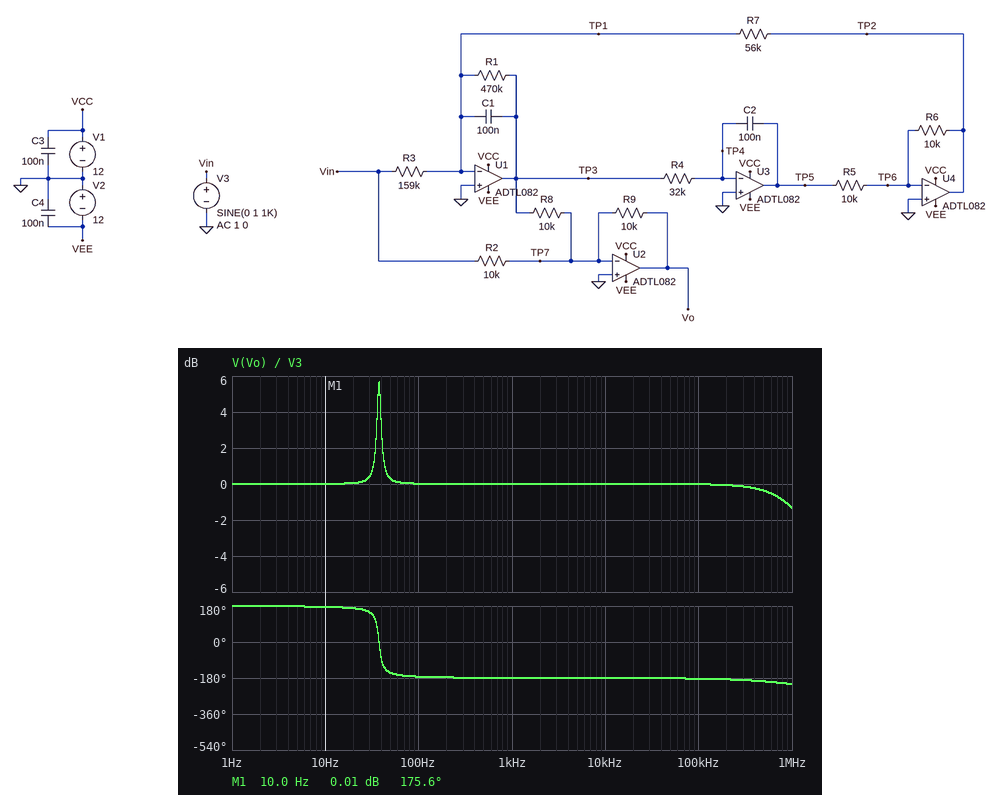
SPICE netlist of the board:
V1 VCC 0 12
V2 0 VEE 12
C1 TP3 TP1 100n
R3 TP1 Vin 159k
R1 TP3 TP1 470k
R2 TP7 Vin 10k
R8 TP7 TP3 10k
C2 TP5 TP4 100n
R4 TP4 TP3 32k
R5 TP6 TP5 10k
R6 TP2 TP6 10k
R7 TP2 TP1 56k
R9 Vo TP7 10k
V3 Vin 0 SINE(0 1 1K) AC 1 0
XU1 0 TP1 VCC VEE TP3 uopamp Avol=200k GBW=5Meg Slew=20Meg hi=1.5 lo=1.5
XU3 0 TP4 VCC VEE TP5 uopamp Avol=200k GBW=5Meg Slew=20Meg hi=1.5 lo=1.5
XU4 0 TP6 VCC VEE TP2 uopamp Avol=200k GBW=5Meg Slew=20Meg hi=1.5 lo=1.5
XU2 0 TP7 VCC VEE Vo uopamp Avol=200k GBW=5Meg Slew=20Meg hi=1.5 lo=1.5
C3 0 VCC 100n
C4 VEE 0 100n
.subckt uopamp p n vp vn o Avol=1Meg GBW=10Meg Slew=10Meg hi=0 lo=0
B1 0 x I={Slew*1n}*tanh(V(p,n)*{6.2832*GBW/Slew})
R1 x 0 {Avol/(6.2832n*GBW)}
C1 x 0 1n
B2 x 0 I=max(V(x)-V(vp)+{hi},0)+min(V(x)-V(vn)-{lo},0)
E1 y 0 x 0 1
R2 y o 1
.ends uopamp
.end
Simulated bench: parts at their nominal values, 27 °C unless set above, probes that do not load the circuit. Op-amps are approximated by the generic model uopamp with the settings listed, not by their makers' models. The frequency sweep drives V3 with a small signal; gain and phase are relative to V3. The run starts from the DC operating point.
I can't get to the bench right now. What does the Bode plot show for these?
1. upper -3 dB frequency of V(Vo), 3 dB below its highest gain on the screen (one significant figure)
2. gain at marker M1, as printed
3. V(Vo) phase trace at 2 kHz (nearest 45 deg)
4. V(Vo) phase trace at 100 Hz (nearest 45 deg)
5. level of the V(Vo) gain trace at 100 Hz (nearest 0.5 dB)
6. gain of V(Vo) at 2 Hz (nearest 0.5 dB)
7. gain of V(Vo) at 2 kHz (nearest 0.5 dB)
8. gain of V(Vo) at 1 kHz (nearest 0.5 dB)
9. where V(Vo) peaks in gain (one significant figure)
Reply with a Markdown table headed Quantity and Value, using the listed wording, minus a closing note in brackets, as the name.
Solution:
| Quantity | Value |
|---|---|
| upper -3 dB frequency of V(Vo), 3 dB below its highest gain on the screen | 40 Hz |
| gain at marker M1, as printed | 0.01 dB |
| V(Vo) phase trace at 2 kHz | -180 deg |
| V(Vo) phase trace at 100 Hz | -180 deg |
| level of the V(Vo) gain trace at 100 Hz | 0 dB |
| gain of V(Vo) at 2 Hz | 0 dB |
| gain of V(Vo) at 2 kHz | 0 dB |
| gain of V(Vo) at 1 kHz | 0 dB |
| where V(Vo) peaks in gain | 40 Hz |
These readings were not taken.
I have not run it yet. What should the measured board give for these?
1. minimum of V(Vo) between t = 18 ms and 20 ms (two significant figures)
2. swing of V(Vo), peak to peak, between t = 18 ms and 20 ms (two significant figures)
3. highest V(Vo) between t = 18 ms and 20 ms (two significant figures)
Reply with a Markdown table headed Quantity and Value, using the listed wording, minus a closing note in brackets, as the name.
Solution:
| Quantity | Value |
|---|---|
| minimum of V(Vo) between t = 18 ms and 20 ms | -1.0 V |
| swing of V(Vo), peak to peak, between t = 18 ms and 20 ms | 2.0 V |
| highest V(Vo) between t = 18 ms and 20 ms | 1.0 V |
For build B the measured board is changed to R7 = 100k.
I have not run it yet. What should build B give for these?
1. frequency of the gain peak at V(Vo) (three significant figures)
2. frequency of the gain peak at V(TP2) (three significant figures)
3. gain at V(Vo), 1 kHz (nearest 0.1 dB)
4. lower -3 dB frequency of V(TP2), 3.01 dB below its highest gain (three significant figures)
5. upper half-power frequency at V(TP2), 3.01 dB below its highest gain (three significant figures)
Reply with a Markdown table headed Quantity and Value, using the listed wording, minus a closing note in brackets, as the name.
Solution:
| Quantity | Value |
|---|---|
| frequency of the gain peak at V(Vo) | 28.1 Hz |
| frequency of the gain peak at V(TP2) | 28.0 Hz |
| gain at V(Vo), 1 kHz | 0 dB |
| lower -3 dB frequency of V(TP2), 3.01 dB below its highest gain | 26.3 Hz |
| upper half-power frequency at V(TP2), 3.01 dB below its highest gain | 29.7 Hz |
